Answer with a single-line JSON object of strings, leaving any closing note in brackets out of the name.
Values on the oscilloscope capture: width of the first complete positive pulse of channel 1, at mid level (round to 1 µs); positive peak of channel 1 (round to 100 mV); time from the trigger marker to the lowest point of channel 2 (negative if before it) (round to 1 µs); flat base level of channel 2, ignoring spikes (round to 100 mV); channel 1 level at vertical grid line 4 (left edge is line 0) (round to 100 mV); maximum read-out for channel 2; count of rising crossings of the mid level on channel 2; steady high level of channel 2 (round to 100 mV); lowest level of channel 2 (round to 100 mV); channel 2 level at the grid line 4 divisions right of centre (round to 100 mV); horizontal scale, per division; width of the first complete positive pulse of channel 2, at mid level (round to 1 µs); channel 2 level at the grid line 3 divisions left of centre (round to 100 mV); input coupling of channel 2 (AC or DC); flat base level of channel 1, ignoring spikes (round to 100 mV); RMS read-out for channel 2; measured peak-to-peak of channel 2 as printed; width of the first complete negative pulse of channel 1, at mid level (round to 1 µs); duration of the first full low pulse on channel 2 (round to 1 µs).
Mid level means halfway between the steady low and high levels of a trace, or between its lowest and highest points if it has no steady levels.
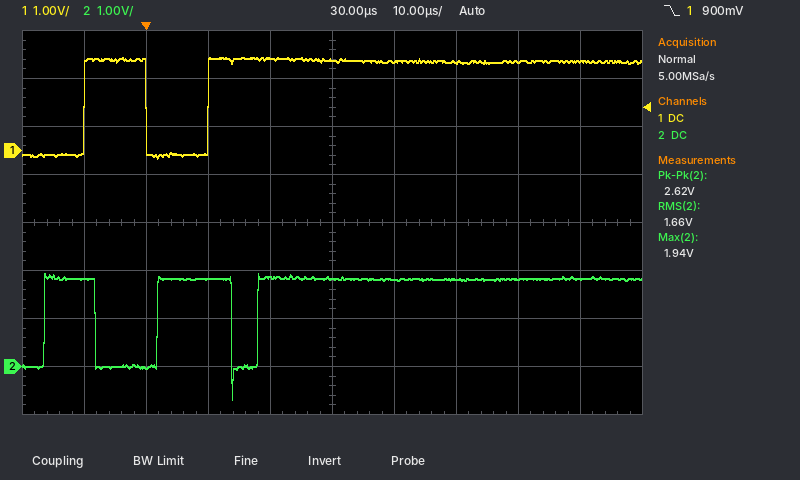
{"width of the first complete positive pulse of channel 1, at mid level": "10 µs", "positive peak of channel 1": "1.9 V", "time from the trigger marker to the lowest point of channel 2 (negative if before it)": "+14 µs", "flat base level of channel 2, ignoring spikes": "0.0 V", "channel 1 level at vertical grid line 4 (left edge is line 0)": "1.9 V", "maximum read-out for channel 2": "1.94 V", "count of rising crossings of the mid level on channel 2": "3", "steady high level of channel 2": "1.8 V", "lowest level of channel 2": "-700 mV", "channel 2 level at the grid line 4 divisions right of centre": "1.8 V", "horizontal scale, per division": "10 µs", "width of the first complete positive pulse of channel 2, at mid level": "8 µs", "channel 2 level at the grid line 3 divisions left of centre": "0.0 V", "input coupling of channel 2": "DC", "flat base level of channel 1, ignoring spikes": "-100 mV", "RMS read-out for channel 2": "1.66 V", "measured peak-to-peak of channel 2 as printed": "2.62 V", "width of the first complete negative pulse of channel 1, at mid level": "10 µs", "duration of the first full low pulse on channel 2": "10 µs"}
